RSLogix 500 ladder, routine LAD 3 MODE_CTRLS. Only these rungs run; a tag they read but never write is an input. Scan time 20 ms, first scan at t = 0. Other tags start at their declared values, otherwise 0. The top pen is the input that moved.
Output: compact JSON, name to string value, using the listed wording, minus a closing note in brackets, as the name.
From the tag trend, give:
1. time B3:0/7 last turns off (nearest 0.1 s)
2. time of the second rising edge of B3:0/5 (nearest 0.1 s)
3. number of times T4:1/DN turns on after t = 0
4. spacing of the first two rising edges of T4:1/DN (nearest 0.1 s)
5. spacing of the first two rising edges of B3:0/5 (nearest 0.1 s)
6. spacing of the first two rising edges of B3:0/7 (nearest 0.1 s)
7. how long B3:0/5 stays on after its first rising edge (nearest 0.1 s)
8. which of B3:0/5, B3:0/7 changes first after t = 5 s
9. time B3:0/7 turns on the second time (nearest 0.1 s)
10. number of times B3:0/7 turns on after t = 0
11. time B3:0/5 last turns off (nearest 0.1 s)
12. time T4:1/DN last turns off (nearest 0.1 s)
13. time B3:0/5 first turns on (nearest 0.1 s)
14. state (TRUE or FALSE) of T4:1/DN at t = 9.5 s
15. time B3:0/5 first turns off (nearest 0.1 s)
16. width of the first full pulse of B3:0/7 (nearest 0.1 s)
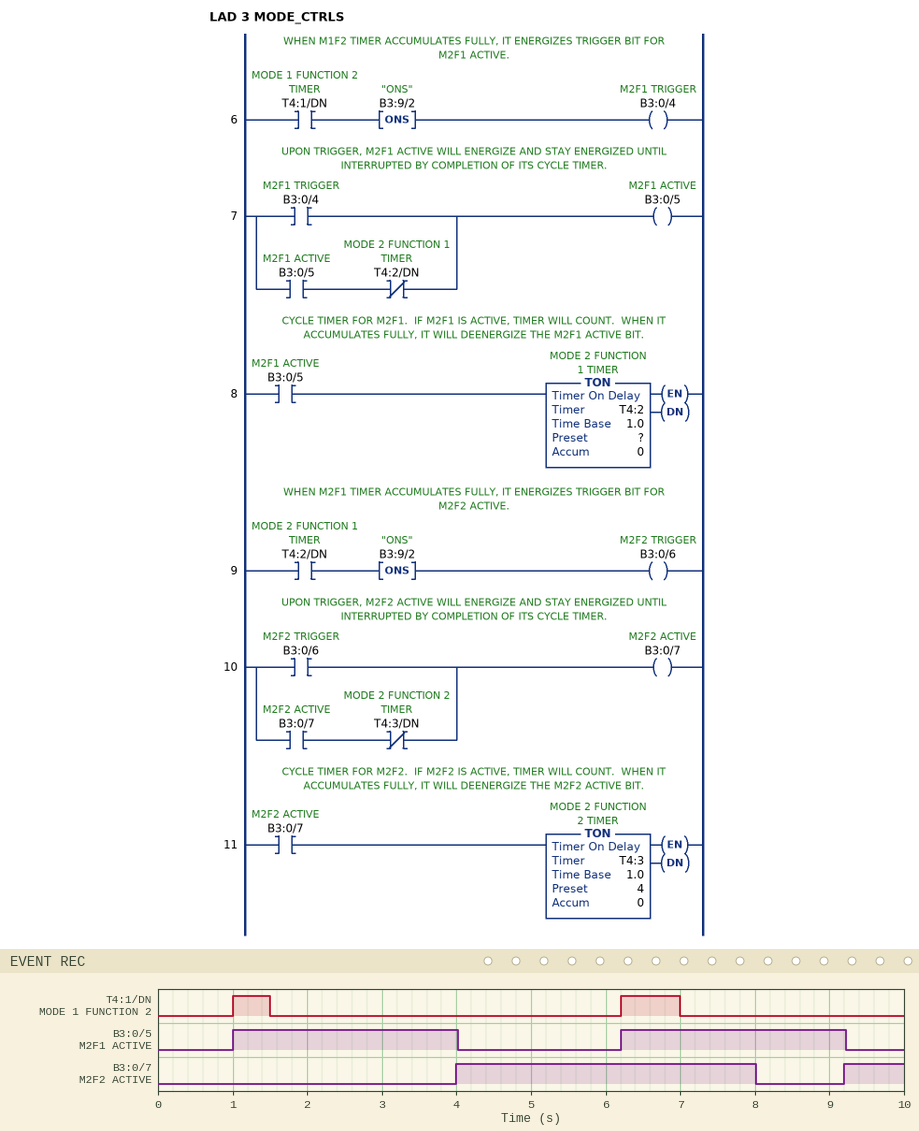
{"time B3:0/7 last turns off": "8.0 s", "time of the second rising edge of B3:0/5": "6.2 s", "number of times T4:1/DN turns on after t = 0": "2", "spacing of the first two rising edges of T4:1/DN": "5.2 s", "spacing of the first two rising edges of B3:0/5": "5.2 s", "spacing of the first two rising edges of B3:0/7": "5.2 s", "how long B3:0/5 stays on after its first rising edge": "3.0 s", "which of B3:0/5, B3:0/7 changes first after t = 5 s": "B3:0/5", "time B3:0/7 turns on the second time": "9.2 s", "number of times B3:0/7 turns on after t = 0": "2", "time B3:0/5 last turns off": "9.2 s", "time T4:1/DN last turns off": "7.0 s", "time B3:0/5 first turns on": "1.0 s", "state (TRUE or FALSE) of T4:1/DN at t = 9.5 s": "FALSE", "time B3:0/5 first turns off": "4.0 s", "width of the first full pulse of B3:0/7": "4.0 s"}
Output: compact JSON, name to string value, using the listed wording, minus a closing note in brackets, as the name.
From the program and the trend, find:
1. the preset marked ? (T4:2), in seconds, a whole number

{"the preset marked ? (T4:2), in seconds, a whole number": "3 s"}
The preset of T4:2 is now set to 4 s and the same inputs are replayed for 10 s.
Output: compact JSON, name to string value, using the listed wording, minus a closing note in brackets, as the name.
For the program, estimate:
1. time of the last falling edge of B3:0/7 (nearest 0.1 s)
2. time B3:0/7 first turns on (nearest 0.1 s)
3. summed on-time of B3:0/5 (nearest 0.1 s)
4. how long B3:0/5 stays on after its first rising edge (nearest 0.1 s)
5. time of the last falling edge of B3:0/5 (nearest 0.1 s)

{"time of the last falling edge of B3:0/7": "9.0 s", "time B3:0/7 first turns on": "5.0 s", "summed on-time of B3:0/5": "7.8 s", "how long B3:0/5 stays on after its first rising edge": "4.0 s", "time of the last falling edge of B3:0/5": "5.0 s"}
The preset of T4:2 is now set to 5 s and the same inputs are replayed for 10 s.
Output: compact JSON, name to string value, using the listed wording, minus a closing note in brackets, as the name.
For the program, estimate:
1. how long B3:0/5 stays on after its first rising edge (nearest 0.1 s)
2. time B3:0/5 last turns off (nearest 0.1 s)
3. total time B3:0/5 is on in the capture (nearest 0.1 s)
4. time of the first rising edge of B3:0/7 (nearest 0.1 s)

{"how long B3:0/5 stays on after its first rising edge": "5.0 s", "time B3:0/5 last turns off": "6.0 s", "total time B3:0/5 is on in the capture": "8.8 s", "time of the first rising edge of B3:0/7": "6.0 s"}
